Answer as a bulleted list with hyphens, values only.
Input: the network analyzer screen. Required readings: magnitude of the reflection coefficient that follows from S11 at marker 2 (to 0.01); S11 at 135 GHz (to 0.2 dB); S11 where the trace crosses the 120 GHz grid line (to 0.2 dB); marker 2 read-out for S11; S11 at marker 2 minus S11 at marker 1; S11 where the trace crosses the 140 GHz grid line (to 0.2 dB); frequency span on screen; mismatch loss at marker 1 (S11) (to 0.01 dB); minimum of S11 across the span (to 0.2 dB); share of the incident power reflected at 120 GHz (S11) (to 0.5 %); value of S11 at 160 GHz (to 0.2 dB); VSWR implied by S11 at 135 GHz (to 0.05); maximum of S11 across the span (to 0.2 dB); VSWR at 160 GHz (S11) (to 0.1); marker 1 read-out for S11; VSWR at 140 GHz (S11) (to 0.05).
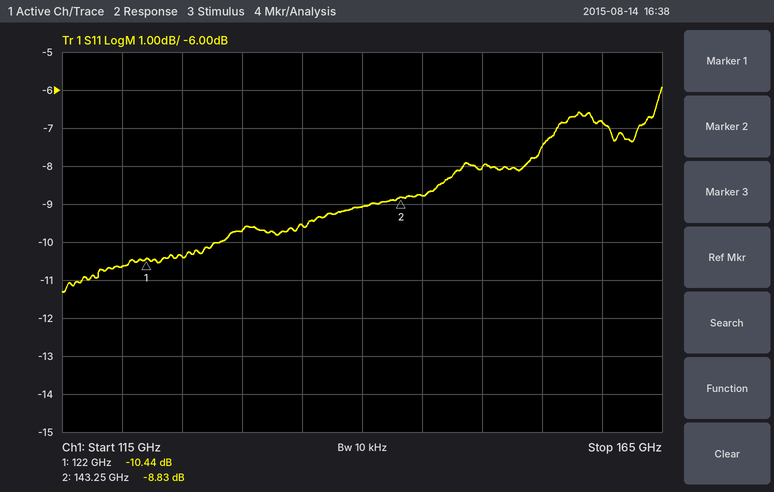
- 0.36
- -9.6 dB
- -10.6 dB
- -8.83 dB
- 1.61 dB
- -9.0 dB
- 50 GHz
- 0.41 dB
- -11.4 dB
- 8.5 %
- -6.8 dB
- 2.00
- -6.0 dB
- 2.7
- -10.44 dB
- 2.10
